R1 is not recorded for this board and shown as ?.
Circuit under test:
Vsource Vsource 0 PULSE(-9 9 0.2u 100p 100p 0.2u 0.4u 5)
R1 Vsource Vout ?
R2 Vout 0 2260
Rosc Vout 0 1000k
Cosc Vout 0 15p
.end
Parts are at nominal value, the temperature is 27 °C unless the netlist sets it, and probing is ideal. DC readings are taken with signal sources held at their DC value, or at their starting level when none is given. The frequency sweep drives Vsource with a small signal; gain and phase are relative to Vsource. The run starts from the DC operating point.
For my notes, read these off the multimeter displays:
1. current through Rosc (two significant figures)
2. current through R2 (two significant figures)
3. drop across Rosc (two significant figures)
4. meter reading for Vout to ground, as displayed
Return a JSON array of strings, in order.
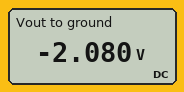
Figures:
["2.1 µA", "920 µA", "2.1 V", "-2.080 V"]
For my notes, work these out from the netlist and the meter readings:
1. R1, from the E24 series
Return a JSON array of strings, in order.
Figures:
["7.5 kΩ"]
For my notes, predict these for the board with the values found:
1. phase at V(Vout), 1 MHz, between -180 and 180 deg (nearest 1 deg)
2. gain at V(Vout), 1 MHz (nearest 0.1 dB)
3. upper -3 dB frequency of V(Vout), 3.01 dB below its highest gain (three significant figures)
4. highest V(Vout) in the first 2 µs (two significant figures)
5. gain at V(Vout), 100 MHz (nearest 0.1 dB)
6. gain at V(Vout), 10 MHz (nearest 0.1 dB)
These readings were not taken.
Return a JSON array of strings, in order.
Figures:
["-9 deg", "-12.8 dB", "6.12 MHz", "2.1 V", "-37.0 dB", "-18.4 dB"]
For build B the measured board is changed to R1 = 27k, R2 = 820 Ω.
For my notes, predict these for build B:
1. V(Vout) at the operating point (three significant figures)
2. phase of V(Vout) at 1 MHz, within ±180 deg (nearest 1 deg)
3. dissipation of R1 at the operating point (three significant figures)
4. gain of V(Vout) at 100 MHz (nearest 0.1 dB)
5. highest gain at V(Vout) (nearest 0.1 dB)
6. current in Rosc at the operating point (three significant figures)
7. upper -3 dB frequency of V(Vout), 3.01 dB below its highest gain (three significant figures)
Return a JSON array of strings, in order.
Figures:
["-265 mV", "-4 deg", "2.83 mW", "-48.2 dB", "-30.6 dB", "265 nA", "13.3 MHz"]
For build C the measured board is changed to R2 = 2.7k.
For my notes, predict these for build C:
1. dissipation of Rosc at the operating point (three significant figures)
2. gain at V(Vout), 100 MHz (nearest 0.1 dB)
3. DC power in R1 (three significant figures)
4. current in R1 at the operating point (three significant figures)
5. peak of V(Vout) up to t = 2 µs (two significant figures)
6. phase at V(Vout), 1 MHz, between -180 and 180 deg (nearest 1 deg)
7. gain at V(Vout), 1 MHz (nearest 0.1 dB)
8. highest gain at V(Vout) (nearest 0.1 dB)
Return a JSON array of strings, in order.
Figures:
["5.65 µW", "-37.0 dB", "5.85 mW", "883 µA", "2.4 V", "-11 deg", "-11.7 dB", "-11.6 dB"]
